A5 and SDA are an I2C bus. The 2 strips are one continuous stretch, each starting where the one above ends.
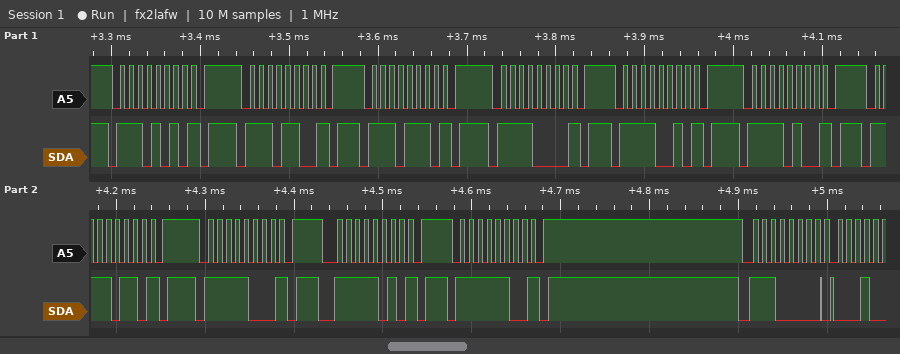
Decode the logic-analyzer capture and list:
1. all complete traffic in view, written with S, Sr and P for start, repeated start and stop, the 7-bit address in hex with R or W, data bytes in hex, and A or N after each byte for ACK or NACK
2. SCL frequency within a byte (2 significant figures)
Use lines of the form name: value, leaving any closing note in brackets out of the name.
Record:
all complete traffic in view, written with S, Sr and P for start, repeated start and stop, the 7-bit address in hex with R or W, data bytes in hex, and A or N after each byte for ACK or NACK: S 75W N P S 76W N P S 77W N P S 78W N P S 79W N P S 7AW N P S 7BW N P S 7CW N P S 7DW N P S 7EW N P S 70W A
SCL frequency within a byte: 100 kHz
